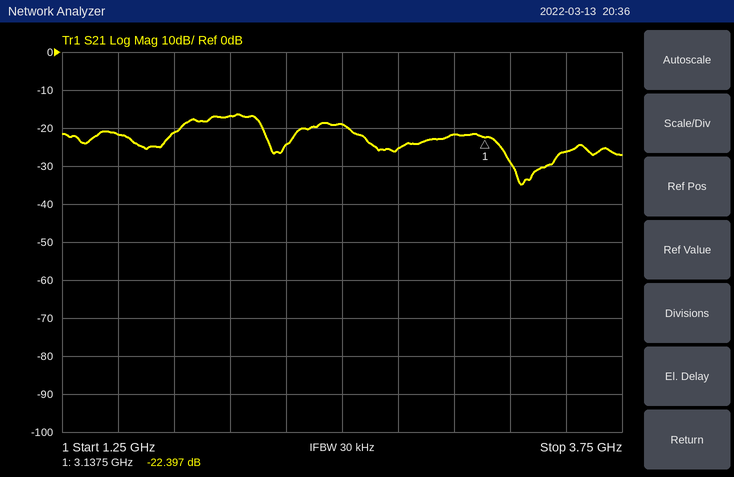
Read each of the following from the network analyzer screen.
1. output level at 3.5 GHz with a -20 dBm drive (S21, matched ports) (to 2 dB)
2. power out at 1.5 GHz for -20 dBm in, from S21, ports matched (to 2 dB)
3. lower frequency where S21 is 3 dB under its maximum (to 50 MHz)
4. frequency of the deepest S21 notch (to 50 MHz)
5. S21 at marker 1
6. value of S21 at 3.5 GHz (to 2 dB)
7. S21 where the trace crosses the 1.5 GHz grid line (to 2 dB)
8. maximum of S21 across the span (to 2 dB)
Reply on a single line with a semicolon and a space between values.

-46 dBm; -42 dBm; 1.80 GHz; 3.30 GHz; -22.397 dB; -26 dB; -22 dB; -16 dB
